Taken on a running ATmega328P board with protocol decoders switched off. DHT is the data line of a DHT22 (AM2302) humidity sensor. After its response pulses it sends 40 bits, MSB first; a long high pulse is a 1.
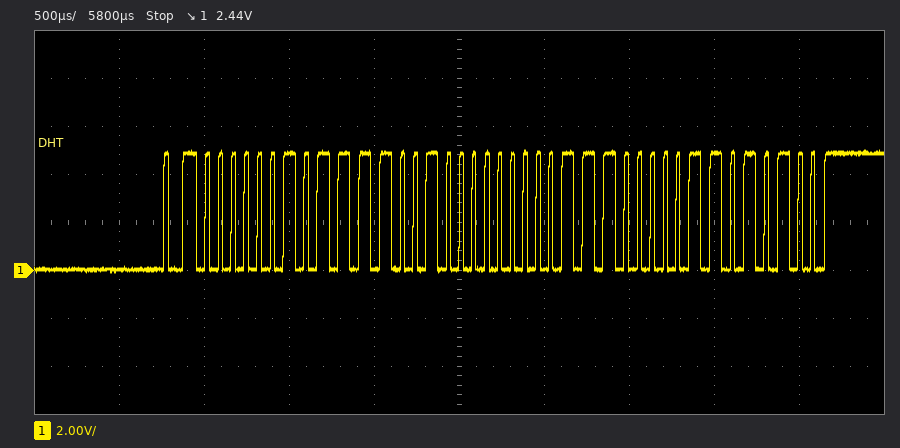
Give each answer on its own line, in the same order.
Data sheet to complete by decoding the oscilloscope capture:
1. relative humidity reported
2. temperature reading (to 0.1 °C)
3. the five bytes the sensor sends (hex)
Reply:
75.4 %
22.4 °C
02 F2 00 E0 D4
